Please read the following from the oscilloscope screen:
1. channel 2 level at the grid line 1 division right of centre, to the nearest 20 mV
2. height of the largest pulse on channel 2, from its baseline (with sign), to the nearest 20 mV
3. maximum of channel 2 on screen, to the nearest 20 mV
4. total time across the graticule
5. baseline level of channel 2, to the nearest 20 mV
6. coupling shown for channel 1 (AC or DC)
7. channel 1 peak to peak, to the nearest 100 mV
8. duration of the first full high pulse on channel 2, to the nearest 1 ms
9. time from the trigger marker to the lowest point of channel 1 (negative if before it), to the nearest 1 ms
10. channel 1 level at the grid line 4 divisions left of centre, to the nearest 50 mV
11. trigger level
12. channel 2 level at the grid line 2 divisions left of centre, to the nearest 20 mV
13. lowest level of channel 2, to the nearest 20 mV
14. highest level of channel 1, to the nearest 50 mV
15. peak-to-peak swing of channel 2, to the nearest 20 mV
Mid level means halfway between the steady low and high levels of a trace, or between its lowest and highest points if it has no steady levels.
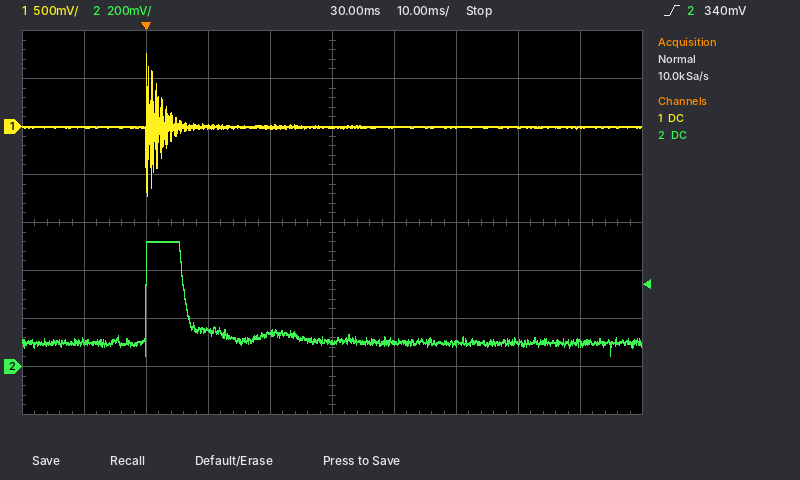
100 mV
+420 mV
520 mV
100 ms
100 mV
DC
1.50 V
6 ms
0 ms
0 mV
340 mV
160 mV
40 mV
750 mV
480 mV
